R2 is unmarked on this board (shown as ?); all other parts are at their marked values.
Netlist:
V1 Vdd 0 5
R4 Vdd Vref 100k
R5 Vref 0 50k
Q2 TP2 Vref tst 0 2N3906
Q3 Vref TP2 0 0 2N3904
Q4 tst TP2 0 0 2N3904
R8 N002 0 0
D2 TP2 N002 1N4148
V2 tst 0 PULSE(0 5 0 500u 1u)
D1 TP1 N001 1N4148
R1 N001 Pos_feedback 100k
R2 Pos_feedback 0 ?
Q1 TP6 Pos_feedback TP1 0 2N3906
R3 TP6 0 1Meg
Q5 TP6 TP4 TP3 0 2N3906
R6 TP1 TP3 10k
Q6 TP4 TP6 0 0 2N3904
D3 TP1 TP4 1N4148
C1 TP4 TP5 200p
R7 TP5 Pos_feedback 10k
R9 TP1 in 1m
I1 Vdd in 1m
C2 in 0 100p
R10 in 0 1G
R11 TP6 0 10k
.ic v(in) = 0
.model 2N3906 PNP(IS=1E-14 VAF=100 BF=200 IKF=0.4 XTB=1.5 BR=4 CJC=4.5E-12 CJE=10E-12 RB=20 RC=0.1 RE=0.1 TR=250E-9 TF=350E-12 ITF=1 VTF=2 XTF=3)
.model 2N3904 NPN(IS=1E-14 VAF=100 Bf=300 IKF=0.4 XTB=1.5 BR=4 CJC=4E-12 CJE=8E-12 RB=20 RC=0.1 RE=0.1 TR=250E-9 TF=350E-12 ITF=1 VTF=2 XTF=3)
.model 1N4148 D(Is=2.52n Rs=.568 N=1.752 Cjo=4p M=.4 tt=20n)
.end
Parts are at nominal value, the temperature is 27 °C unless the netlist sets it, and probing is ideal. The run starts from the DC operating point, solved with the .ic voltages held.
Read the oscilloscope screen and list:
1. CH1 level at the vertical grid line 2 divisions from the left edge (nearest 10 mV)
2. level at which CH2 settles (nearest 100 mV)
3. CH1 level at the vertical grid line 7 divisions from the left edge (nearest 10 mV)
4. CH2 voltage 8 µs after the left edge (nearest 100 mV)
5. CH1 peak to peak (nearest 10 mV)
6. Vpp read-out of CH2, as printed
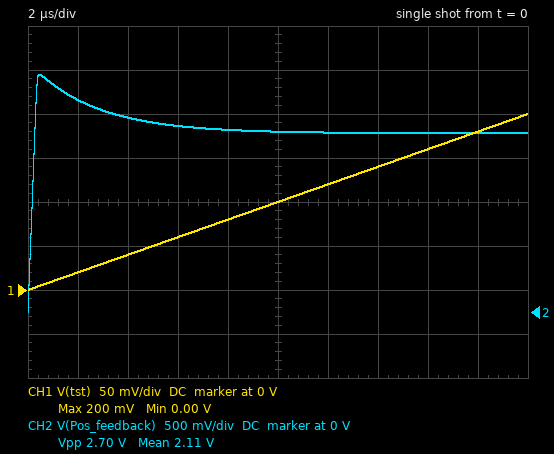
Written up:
40 mV
2.0 V
140 mV
2.1 V
200 mV
2.70 V
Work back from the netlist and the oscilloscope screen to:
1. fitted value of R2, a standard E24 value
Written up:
680 kΩ
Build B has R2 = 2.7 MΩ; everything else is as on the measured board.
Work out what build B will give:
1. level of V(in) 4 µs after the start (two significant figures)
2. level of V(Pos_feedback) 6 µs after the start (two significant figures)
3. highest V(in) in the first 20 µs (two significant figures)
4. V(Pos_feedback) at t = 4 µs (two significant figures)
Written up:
5.7 V
5.9 V
8.3 V
5.1 V
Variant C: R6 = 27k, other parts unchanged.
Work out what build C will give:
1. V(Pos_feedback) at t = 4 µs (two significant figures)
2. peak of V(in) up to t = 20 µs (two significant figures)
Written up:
2.3 V
3.2 V
